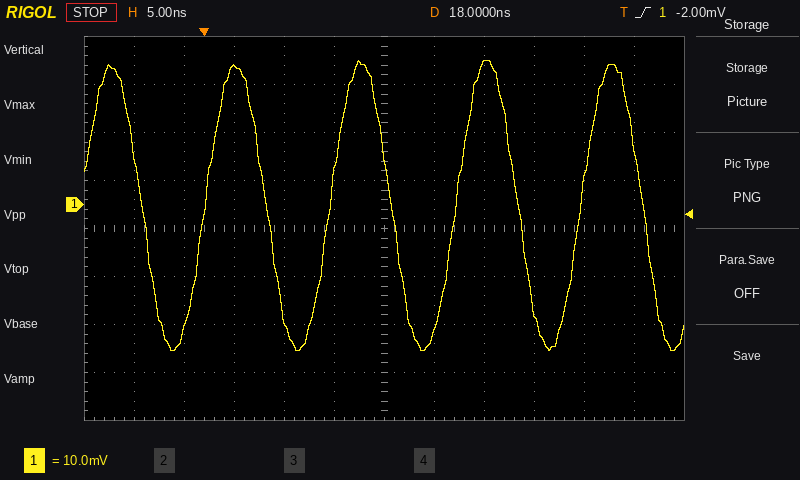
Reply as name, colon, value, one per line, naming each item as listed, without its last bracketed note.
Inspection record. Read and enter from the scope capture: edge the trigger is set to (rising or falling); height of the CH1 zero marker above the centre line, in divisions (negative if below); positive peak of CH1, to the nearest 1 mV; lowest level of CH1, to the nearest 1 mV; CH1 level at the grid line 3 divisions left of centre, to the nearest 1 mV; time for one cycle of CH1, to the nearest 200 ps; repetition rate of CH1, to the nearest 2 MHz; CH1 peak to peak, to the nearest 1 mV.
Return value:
edge the trigger is set to: rising
height of the CH1 zero marker above the centre line, in divisions: +0.5 div
positive peak of CH1, to the nearest 1 mV: 30 mV
lowest level of CH1, to the nearest 1 mV: -30 mV
CH1 level at the grid line 3 divisions left of centre, to the nearest 1 mV: 29 mV
time for one cycle of CH1, to the nearest 200 ps: 12.6 ns
repetition rate of CH1, to the nearest 2 MHz: 80 MHz
CH1 peak to peak, to the nearest 1 mV: 60 mV
